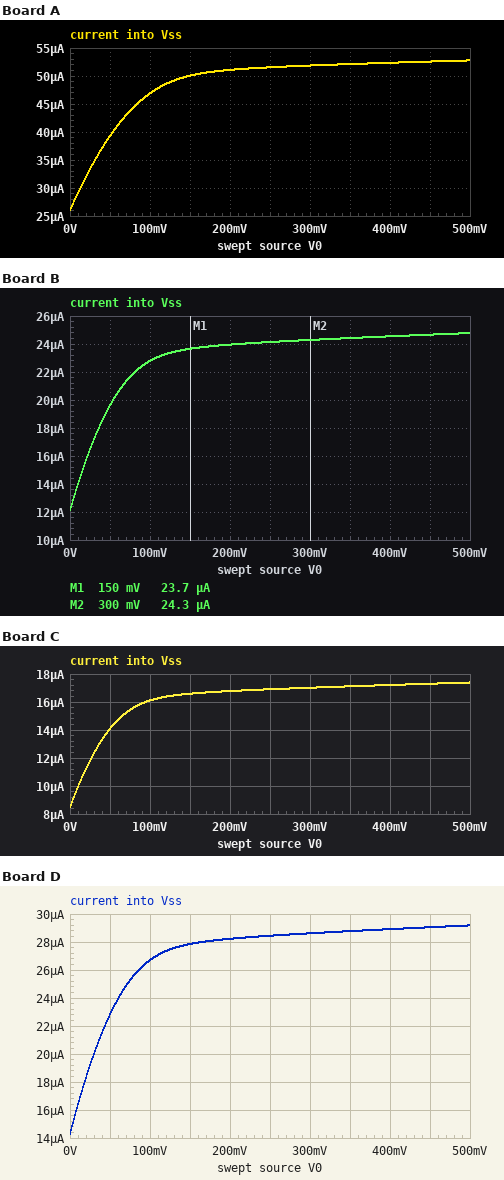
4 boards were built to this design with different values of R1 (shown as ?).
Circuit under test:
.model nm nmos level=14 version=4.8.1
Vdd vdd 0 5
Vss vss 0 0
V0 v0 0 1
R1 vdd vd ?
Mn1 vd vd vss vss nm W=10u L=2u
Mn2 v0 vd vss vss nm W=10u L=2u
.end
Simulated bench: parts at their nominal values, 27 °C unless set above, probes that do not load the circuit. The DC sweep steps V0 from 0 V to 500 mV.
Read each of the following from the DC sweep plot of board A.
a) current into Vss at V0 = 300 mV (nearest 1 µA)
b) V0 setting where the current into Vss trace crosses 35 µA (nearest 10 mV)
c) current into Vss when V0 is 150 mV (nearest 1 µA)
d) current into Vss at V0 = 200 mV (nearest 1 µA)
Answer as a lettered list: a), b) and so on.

a) 52 µA
b) 30 mV
c) 50 µA
d) 51 µA
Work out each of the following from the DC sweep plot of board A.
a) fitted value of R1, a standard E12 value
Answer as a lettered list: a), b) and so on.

a) 180 kΩ
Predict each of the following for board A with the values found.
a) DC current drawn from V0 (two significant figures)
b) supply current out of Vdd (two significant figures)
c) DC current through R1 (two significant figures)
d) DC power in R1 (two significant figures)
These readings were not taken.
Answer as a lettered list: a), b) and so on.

a) 29 µA
b) 26 µA
c) 26 µA
d) 120 µW
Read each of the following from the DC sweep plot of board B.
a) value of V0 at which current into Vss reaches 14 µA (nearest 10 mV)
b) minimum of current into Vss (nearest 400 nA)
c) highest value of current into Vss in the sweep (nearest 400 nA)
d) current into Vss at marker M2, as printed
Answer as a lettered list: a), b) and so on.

a) 10 mV
b) 12.0 µA
c) 24.8 µA
d) 24.3 µA
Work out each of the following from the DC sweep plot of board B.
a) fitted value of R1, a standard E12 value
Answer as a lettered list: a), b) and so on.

a) 390 kΩ
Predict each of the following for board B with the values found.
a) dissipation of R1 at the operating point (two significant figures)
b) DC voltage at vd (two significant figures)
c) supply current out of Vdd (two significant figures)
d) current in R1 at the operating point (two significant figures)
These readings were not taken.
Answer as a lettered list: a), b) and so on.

a) 57 µW
b) 280 mV
c) 12 µA
d) 12 µA
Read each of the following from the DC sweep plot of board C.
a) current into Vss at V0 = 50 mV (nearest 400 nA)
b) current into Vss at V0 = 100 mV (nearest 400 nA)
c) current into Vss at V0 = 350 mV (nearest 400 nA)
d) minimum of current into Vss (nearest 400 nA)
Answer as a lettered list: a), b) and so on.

a) 14.0 µA
b) 16.0 µA
c) 17.2 µA
d) 8.4 µA
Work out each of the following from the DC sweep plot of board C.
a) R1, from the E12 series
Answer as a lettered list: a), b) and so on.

a) 560 kΩ
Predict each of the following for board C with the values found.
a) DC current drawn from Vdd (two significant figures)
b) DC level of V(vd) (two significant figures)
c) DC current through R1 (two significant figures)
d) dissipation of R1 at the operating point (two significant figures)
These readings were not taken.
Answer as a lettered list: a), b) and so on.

a) 8.5 µA
b) 260 mV
c) 8.5 µA
d) 40 µW
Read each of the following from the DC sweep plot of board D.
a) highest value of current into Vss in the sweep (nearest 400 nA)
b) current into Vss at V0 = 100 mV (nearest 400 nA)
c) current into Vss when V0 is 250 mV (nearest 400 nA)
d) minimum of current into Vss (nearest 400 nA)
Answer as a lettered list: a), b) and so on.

a) 29.2 µA
b) 26.8 µA
c) 28.4 µA
d) 14.4 µA
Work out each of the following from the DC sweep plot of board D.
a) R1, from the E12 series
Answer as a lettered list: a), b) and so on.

a) 330 kΩ
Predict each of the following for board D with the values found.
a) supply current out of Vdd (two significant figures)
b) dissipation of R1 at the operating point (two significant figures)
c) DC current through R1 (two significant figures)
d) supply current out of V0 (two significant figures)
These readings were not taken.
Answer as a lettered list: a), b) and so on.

a) 14 µA
b) 67 µW
c) 14 µA
d) 16 µA
